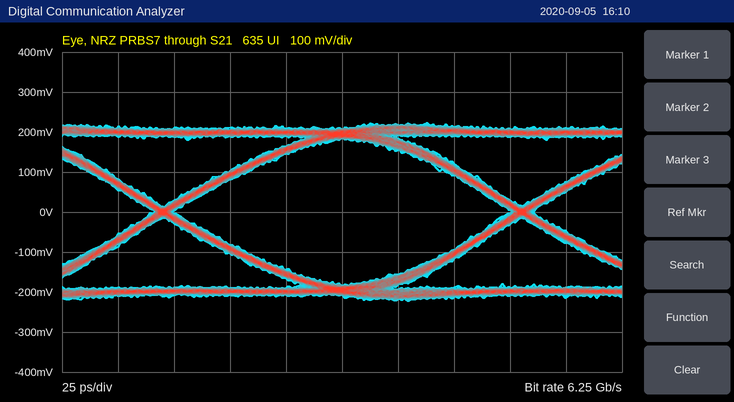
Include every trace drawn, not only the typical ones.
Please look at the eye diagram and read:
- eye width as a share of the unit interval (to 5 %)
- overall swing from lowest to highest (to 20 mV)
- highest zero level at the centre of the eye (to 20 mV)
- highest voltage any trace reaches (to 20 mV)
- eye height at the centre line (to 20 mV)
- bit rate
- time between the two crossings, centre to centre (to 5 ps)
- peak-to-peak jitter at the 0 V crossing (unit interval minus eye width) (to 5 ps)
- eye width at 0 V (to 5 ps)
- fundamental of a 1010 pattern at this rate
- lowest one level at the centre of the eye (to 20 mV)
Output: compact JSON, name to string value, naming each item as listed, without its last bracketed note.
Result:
{"eye width as a share of the unit interval": "95 %", "overall swing from lowest to highest": "440 mV", "highest zero level at the centre of the eye": "-180 mV", "highest voltage any trace reaches": "220 mV", "eye height at the centre line": "360 mV", "bit rate": "6.25 Gb/s", "time between the two crossings, centre to centre": "160 ps", "peak-to-peak jitter at the 0 V crossing (unit interval minus eye width)": "10 ps", "eye width at 0 V": "150 ps", "fundamental of a 1010 pattern at this rate": "3.125 GHz", "lowest one level at the centre of the eye": "180 mV"}
